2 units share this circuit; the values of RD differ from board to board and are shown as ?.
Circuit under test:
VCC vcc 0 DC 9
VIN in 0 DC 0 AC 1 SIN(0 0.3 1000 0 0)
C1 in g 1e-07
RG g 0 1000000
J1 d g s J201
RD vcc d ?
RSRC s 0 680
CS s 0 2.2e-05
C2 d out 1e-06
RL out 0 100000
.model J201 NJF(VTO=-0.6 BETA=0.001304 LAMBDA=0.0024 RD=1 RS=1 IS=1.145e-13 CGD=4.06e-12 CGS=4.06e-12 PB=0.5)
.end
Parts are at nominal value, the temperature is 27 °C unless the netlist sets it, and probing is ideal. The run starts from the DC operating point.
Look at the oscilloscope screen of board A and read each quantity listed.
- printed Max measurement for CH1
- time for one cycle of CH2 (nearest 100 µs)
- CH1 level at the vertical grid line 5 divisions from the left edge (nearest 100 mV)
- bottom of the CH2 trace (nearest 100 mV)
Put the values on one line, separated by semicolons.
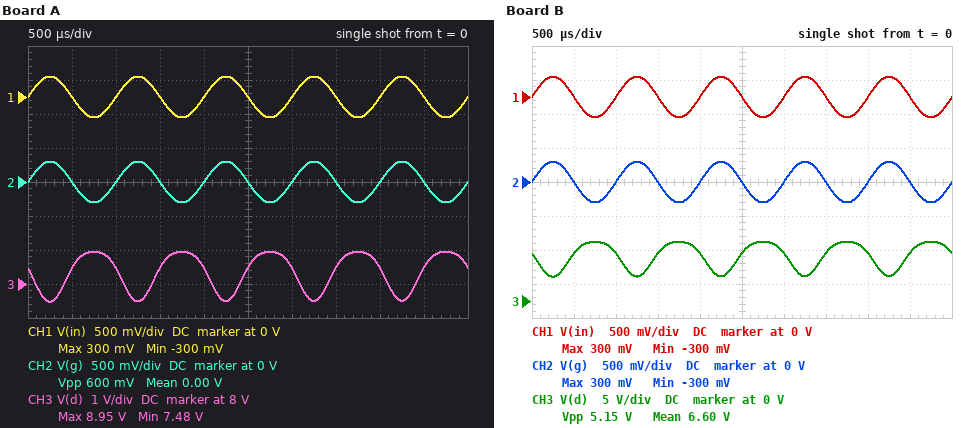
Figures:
300 mV; 1.0 ms; 0 V; -300 mV
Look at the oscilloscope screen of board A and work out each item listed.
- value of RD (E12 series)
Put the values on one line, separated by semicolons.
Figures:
2.2 kΩ
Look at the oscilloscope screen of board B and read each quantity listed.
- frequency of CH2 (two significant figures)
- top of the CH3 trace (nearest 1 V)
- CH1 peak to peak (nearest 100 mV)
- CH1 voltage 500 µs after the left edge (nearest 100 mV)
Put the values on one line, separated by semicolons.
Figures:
1.0 kHz; 9 V; 600 mV; 0 V
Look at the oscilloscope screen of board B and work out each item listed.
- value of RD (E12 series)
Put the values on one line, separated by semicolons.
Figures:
8.2 kΩ
